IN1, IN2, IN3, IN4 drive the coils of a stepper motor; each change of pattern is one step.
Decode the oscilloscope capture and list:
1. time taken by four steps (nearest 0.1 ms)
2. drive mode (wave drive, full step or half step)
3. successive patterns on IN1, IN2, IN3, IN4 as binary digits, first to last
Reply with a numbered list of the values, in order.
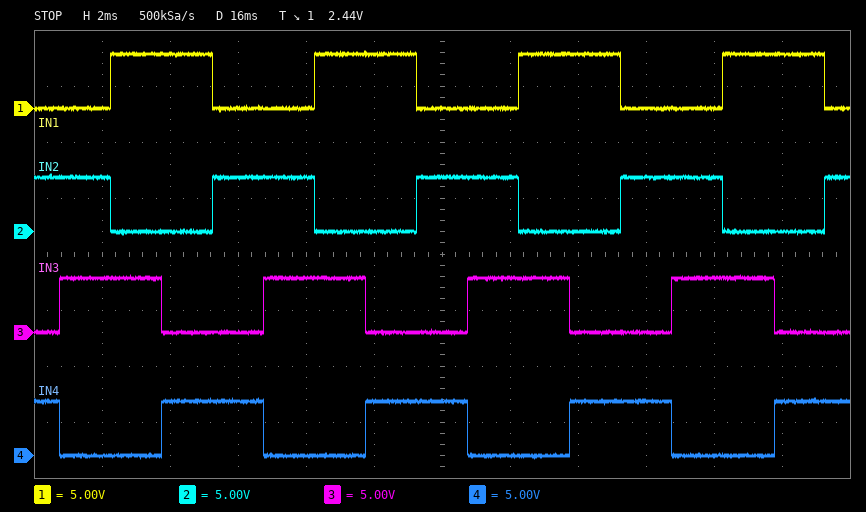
1. 6.0 ms
2. full step
3. 0101 0110 1010 1001 0101 0110 1010 1001 0101 0110 1010 1001 0101 0110 1010 1001 0101
